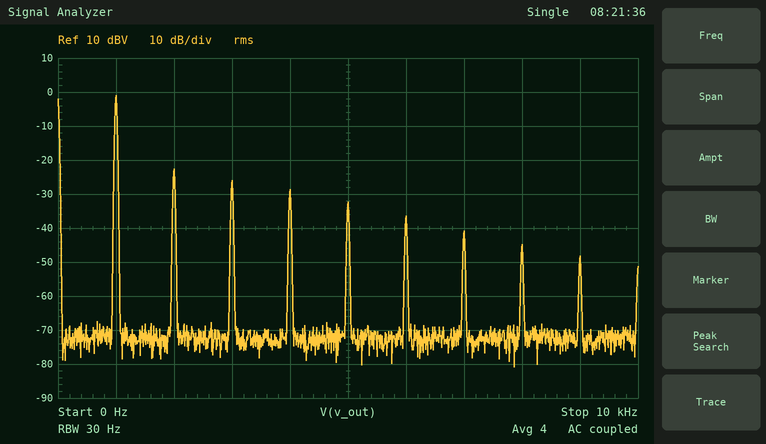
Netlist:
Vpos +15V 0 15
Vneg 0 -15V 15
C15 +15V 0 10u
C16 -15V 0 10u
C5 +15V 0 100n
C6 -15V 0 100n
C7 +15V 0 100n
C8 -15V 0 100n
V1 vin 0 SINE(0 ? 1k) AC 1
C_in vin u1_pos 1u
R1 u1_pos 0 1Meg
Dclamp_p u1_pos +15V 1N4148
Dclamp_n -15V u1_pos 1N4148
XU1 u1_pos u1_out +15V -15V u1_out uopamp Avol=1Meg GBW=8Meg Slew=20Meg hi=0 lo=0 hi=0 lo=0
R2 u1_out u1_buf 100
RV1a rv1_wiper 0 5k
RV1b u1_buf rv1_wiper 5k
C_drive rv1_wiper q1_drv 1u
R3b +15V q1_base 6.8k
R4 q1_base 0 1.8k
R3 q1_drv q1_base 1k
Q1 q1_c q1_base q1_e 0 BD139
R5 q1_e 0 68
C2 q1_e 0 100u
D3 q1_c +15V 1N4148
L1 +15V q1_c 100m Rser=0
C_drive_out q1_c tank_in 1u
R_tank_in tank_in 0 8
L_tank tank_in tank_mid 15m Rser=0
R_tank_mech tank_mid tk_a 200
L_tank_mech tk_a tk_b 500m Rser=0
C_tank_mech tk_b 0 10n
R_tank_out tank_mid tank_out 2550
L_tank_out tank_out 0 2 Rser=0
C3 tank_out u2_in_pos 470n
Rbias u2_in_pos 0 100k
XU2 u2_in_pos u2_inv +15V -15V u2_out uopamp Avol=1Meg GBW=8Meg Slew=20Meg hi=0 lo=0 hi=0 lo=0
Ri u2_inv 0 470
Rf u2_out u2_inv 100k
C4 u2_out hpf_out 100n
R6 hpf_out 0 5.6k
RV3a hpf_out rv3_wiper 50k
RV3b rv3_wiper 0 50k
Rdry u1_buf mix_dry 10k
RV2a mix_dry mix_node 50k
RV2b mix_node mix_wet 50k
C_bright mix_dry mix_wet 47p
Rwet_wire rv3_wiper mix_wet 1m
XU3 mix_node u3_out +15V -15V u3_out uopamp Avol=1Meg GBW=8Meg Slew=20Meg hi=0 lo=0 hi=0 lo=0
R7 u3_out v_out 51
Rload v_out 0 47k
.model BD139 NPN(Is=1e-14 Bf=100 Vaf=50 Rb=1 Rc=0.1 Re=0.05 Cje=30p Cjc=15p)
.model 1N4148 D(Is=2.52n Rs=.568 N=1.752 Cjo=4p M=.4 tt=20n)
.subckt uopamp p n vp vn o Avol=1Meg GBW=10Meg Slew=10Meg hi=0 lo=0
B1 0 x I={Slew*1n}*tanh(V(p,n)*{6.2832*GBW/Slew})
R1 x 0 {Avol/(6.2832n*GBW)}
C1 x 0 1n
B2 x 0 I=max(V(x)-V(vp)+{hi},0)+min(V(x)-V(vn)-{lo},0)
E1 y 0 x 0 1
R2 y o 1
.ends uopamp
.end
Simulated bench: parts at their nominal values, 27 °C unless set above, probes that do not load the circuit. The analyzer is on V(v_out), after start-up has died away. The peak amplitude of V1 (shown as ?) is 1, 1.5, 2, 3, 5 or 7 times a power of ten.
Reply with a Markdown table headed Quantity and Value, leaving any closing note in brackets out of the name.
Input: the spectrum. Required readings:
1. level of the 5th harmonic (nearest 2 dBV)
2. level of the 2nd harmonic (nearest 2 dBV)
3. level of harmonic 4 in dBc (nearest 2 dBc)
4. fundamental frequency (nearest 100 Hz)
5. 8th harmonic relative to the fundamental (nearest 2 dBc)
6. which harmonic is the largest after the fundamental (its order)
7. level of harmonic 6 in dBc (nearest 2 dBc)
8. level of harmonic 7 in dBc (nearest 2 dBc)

| Quantity | Value |
|---|---|
| level of the 5th harmonic | -32 dBV |
| level of the 2nd harmonic | -22 dBV |
| level of harmonic 4 in dBc | -28 dBc |
| fundamental frequency | 1.0 kHz |
| 8th harmonic relative to the fundamental | -44 dBc |
| which harmonic is the largest after the fundamental | 2 |
| level of harmonic 6 in dBc | -36 dBc |
| level of harmonic 7 in dBc | -40 dBc |
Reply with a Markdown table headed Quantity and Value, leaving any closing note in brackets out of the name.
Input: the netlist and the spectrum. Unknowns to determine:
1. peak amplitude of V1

| Quantity | Value |
|---|---|
| peak amplitude of V1 | 200 mV |
